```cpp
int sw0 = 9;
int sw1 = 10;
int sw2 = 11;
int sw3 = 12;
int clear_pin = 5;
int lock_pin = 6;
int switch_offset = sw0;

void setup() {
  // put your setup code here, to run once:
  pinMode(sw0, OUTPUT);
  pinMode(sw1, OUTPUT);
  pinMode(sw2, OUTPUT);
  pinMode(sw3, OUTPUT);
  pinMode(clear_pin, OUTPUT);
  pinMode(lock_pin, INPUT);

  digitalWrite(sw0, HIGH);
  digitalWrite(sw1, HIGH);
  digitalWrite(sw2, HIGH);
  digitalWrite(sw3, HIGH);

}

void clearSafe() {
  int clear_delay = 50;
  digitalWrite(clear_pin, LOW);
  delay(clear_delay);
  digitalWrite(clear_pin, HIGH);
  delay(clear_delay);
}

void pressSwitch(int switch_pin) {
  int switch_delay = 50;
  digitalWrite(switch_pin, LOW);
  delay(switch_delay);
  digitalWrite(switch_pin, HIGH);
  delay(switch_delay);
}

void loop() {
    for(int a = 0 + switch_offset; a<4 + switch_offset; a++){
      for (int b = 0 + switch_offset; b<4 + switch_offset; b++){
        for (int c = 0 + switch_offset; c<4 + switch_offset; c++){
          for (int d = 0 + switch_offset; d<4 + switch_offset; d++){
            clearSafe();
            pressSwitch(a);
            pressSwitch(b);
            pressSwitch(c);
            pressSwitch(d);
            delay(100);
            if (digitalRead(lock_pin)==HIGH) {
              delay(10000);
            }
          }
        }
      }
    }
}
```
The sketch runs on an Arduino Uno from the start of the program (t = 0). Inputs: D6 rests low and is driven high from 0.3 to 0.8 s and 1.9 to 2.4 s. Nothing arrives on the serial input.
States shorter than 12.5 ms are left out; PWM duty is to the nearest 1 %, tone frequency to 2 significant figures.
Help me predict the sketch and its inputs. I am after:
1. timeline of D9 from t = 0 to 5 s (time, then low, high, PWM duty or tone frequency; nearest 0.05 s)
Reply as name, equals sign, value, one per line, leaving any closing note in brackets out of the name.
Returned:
timeline of D9 from t = 0 to 5 s = 0 s high; 0.1 s low; 0.15 s high; 0.2 s low; 0.25 s high; 0.3 s low; 0.35 s high; 0.4 s low; 0.45 s high
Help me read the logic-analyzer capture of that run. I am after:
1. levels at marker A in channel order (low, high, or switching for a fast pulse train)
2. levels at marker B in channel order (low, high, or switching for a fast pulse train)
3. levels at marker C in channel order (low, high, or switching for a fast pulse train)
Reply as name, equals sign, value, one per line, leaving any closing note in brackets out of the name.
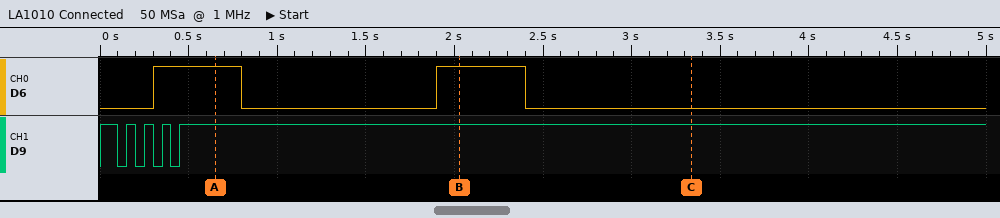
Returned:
levels at marker A in channel order = D6 high, D9 high
levels at marker B in channel order = D6 high, D9 high
levels at marker C in channel order = D6 low, D9 high
